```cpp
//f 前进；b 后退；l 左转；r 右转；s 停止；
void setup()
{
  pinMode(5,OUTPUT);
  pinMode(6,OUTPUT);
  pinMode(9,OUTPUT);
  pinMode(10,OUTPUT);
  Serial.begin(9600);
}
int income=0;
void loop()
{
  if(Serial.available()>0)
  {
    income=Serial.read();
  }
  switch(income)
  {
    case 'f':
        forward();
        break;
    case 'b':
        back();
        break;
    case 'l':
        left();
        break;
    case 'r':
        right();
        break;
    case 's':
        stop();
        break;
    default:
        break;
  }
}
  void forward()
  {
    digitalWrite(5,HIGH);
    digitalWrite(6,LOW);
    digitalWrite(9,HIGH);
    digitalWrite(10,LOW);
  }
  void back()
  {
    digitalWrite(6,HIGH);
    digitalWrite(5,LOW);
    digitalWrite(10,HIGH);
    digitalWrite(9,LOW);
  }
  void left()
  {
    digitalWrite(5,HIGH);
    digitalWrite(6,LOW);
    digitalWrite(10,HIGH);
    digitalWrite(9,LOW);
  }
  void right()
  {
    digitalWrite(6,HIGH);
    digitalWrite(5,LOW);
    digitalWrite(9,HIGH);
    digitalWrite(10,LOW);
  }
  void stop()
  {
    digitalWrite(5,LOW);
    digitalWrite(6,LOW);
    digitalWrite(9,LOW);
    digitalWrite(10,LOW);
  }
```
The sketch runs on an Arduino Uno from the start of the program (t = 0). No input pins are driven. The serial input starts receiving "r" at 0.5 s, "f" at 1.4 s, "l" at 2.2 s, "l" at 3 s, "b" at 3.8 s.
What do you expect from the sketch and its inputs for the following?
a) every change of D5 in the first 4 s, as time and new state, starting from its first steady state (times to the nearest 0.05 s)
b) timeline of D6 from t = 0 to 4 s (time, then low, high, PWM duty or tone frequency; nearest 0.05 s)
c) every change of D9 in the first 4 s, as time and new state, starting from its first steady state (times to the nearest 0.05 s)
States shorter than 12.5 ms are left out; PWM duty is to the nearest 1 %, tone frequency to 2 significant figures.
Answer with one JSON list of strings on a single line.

["0 s low; 1.4 s high; 3.8 s low", "0 s low; 0.5 s high; 1.4 s low; 3.8 s high", "0 s low; 0.5 s high; 2.2 s low"]
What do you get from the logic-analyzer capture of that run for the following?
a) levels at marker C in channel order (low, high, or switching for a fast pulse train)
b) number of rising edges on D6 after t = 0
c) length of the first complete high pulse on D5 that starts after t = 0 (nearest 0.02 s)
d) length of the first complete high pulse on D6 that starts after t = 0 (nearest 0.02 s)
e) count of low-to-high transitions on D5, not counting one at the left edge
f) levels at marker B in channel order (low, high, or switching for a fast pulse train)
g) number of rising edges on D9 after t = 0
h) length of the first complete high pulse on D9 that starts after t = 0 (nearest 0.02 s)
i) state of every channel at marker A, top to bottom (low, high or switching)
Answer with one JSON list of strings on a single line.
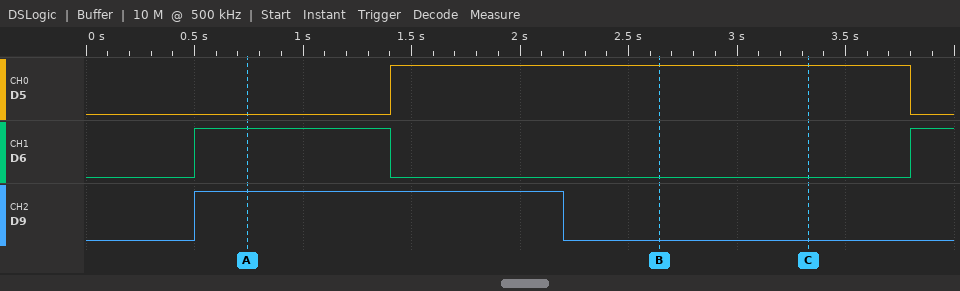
["D5 high, D6 low, D9 low", "2", "2.40 s", "0.90 s", "1", "D5 high, D6 low, D9 low", "1", "1.70 s", "D5 low, D6 high, D9 high"]
